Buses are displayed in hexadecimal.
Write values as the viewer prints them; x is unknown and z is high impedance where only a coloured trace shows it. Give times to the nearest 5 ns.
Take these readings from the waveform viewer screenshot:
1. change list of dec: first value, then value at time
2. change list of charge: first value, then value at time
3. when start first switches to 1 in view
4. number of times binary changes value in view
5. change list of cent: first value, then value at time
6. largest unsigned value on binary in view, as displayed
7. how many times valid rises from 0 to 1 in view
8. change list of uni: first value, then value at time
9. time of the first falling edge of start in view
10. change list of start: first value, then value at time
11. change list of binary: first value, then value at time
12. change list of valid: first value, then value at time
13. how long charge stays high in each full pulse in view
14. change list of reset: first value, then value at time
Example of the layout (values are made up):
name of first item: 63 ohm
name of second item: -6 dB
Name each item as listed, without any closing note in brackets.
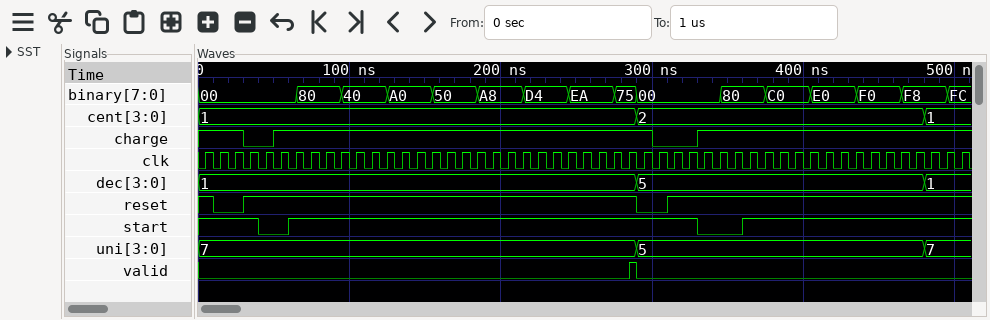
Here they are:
change list of dec: first value, then value at time: 1, 5 at 290 ns, 1 at 480 ns
change list of charge: first value, then value at time: 1, 0 at 30 ns, 1 at 50 ns, 0 at 300 ns, 1 at 330 ns
when start first switches to 1 in view: 60 ns
number of times binary changes value in view: 15
change list of cent: first value, then value at time: 1, 2 at 290 ns, 1 at 480 ns
largest unsigned value on binary in view, as displayed: FC
how many times valid rises from 0 to 1 in view: 1
change list of uni: first value, then value at time: 7, 5 at 290 ns, 7 at 480 ns
time of the first falling edge of start in view: 40 ns
change list of start: first value, then value at time: 1, 0 at 40 ns, 1 at 60 ns, 0 at 330 ns, 1 at 360 ns
change list of binary: first value, then value at time: 00, 80 at 65 ns, 40 at 95 ns, A0 at 125 ns, 50 at 155 ns, A8 at 185 ns, D4 at 215 ns, EA at 245 ns, 75 at 275 ns, 00 at 290 ns, 80 at 345 ns, C0 at 375 ns, E0 at 405 ns, F0 at 435 ns, F8 at 465 ns, FC at 495 ns
change list of valid: first value, then value at time: 0, 1 at 285 ns, 0 at 290 ns
how long charge stays high in each full pulse in view: 250 ns
change list of reset: first value, then value at time: 1, 0 at 10 ns, 1 at 30 ns, 0 at 290 ns, 1 at 310 ns
